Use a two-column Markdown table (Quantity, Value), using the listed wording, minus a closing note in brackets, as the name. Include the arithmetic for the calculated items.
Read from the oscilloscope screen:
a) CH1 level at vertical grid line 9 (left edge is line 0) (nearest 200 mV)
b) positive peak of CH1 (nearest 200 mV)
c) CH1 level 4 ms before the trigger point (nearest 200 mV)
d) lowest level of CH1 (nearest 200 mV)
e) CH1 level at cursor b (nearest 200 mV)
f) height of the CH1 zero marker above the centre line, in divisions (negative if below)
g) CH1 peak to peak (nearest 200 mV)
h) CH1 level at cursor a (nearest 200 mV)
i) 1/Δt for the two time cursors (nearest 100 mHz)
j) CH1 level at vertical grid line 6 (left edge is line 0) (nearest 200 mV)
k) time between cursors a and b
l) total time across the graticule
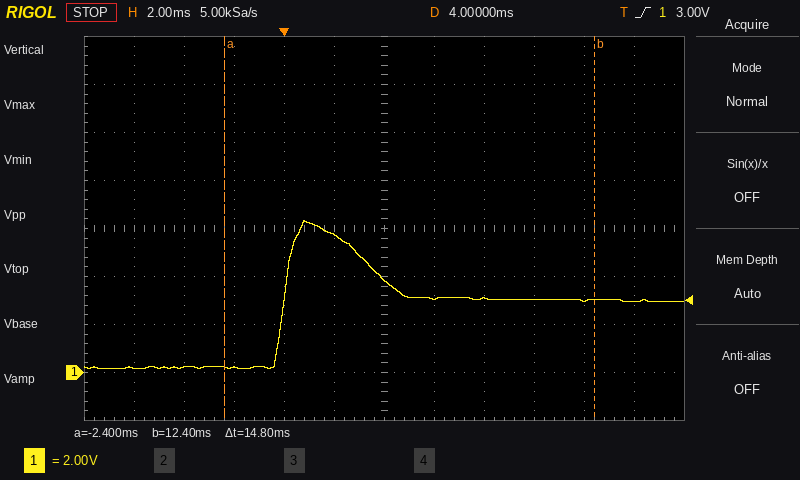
| Quantity | Value |
|---|---|
| CH1 level at vertical grid line 9 (left edge is line 0) | 3.0 V |
| positive peak of CH1 | 6.4 V |
| CH1 level 4 ms before the trigger point | 200 mV |
| lowest level of CH1 | 200 mV |
| CH1 level at cursor b | 3.0 V |
| height of the CH1 zero marker above the centre line, in divisions | -3.0 div |
| CH1 peak to peak | 6.4 V − (200 mV) = 6.2 V |
| CH1 level at cursor a | 200 mV |
| 1/Δt for the two time cursors | 1 / 14.8 ms ≈ 67.6 Hz |
| CH1 level at vertical grid line 6 (left edge is line 0) | 3.8 V |
| time between cursors a and b | 14.8 ms |
| total time across the graticule | 24 ms |
